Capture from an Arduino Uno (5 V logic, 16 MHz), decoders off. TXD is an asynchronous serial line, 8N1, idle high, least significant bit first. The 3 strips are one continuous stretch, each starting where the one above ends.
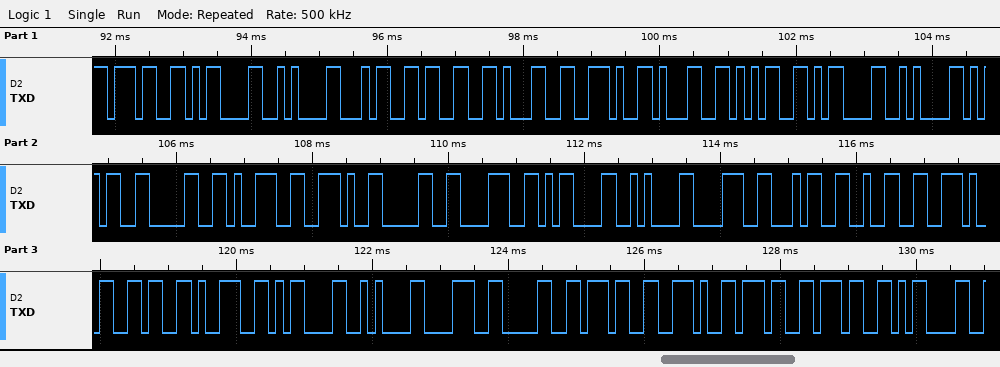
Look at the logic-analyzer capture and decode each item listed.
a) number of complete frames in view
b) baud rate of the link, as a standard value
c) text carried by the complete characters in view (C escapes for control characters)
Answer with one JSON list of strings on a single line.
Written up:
["34", "9600 baud", "\"7\\r\\n431.15\\r\\n509.08\\r\\n842.69\\r\\n807.77\\r\""]
